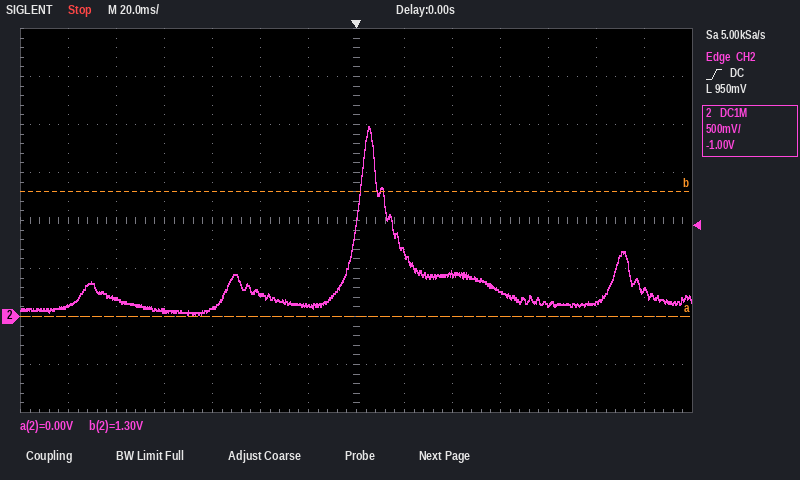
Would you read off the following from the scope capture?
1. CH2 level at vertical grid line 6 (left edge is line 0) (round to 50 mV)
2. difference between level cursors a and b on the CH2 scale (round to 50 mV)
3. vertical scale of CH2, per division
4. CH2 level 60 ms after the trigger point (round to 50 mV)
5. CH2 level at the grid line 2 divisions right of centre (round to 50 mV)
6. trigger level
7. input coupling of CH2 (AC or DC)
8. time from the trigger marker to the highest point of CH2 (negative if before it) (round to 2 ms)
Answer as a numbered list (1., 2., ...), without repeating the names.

1. 100 mV
2. 1.30 V
3. 500 mV
4. 250 mV
5. 450 mV
6. 950 mV
7. DC
8. +6 ms
